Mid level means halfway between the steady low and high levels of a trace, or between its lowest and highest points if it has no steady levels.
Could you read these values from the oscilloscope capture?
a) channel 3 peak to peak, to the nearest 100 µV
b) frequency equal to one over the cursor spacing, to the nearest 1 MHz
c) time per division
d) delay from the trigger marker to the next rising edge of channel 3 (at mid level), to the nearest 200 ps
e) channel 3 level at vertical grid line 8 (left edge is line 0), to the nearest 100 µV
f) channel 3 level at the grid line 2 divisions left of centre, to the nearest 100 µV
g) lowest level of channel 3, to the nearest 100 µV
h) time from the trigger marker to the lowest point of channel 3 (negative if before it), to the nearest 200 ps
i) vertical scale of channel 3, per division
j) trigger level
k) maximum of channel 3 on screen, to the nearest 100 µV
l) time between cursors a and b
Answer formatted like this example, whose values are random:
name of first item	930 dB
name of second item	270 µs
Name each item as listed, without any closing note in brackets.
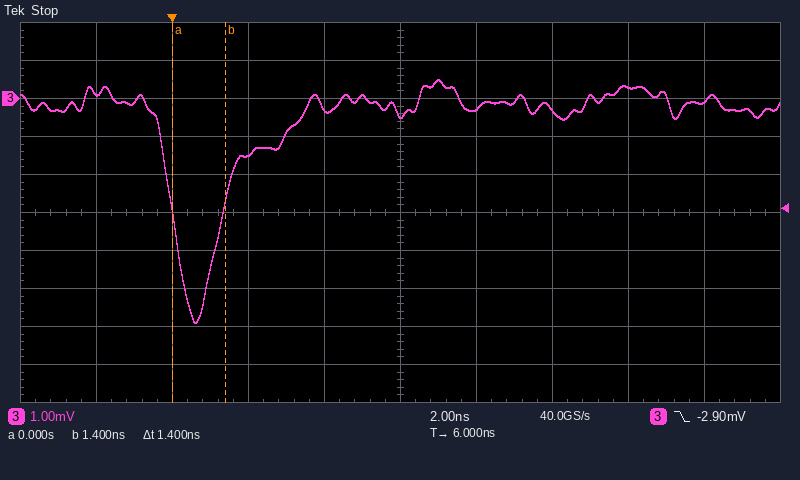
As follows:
channel 3 peak to peak, to the nearest 100 µV	6.4 mV
frequency equal to one over the cursor spacing, to the nearest 1 MHz	714 MHz
time per division	2 ns
delay from the trigger marker to the next rising edge of channel 3 (at mid level), to the nearest 200 ps	1.4 ns
channel 3 level at vertical grid line 8 (left edge is line 0), to the nearest 100 µV	300 µV
channel 3 level at the grid line 2 divisions left of centre, to the nearest 100 µV	-1.5 mV
lowest level of channel 3, to the nearest 100 µV	-5.9 mV
time from the trigger marker to the lowest point of channel 3 (negative if before it), to the nearest 200 ps	+600 ps
vertical scale of channel 3, per division	1 mV
trigger level	-2.90 mV
maximum of channel 3 on screen, to the nearest 100 µV	500 µV
time between cursors a and b	1.4 ns
